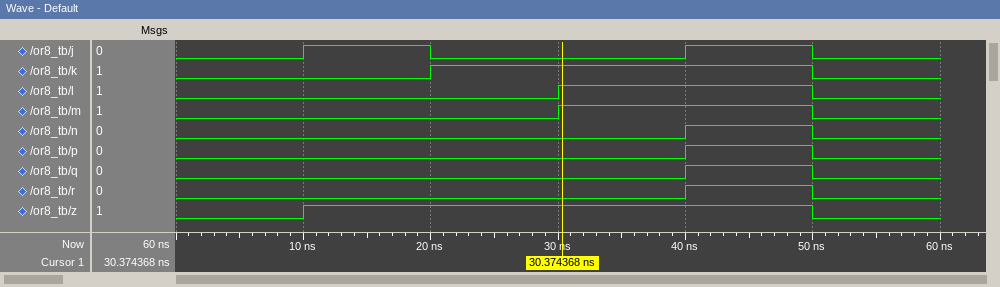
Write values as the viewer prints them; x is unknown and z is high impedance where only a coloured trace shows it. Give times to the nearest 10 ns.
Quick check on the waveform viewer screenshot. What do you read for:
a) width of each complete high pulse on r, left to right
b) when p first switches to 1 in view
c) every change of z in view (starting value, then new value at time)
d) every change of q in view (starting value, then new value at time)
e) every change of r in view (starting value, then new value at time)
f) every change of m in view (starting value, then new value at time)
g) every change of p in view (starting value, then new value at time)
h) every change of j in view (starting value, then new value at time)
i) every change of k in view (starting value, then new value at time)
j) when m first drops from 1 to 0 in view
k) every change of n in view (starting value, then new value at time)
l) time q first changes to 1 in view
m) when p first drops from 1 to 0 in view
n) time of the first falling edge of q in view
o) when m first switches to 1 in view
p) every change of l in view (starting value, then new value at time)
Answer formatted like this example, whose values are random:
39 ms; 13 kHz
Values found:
10 ns; 40 ns; 0, 1 at 10 ns, 0 at 50 ns; 0, 1 at 40 ns, 0 at 50 ns; 0, 1 at 40 ns, 0 at 50 ns; 0, 1 at 30 ns, 0 at 50 ns; 0, 1 at 40 ns, 0 at 50 ns; 0, 1 at 10 ns, 0 at 20 ns, 1 at 40 ns, 0 at 50 ns; 0, 1 at 20 ns, 0 at 50 ns; 50 ns; 0, 1 at 40 ns, 0 at 50 ns; 40 ns; 50 ns; 50 ns; 30 ns; 0, 1 at 30 ns, 0 at 50 ns
